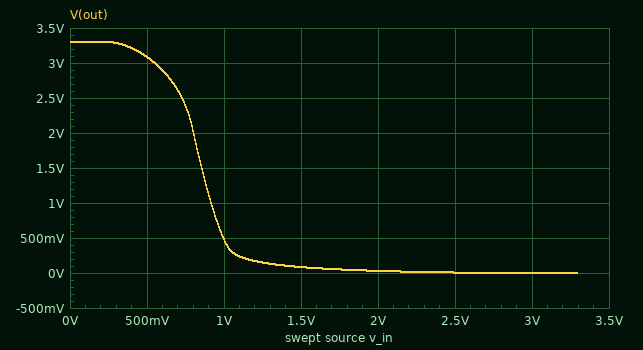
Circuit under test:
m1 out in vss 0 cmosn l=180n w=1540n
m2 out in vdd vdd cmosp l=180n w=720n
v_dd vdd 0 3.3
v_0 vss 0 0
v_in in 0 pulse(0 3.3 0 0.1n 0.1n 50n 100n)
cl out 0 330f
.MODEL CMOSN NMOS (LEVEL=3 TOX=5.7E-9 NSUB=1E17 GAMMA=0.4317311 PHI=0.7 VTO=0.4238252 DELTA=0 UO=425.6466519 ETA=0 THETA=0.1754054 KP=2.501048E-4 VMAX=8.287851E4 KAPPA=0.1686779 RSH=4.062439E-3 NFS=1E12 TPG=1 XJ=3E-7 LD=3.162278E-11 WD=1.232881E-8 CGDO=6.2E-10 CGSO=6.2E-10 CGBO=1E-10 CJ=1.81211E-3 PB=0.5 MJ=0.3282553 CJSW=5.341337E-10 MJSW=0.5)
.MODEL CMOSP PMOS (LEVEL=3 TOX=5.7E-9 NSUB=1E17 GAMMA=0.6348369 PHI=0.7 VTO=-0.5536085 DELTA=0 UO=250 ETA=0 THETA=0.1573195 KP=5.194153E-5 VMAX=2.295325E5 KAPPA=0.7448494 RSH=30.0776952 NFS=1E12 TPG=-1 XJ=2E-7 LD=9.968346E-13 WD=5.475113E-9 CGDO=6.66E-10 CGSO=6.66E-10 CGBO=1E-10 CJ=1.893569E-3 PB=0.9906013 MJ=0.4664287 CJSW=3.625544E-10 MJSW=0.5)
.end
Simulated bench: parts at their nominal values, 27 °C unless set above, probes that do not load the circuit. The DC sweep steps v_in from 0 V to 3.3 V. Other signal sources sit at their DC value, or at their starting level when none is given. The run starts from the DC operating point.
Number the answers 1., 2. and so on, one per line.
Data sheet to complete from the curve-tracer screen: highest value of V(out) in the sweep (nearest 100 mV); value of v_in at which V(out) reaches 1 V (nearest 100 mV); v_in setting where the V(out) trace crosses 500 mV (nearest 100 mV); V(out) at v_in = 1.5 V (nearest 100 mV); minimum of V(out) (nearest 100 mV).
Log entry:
1. 3.3 V
2. 900 mV
3. 1.0 V
4. 100 mV
5. 0 V
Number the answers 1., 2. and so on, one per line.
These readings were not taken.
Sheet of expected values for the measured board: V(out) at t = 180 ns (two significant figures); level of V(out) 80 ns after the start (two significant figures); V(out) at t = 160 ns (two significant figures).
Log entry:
1. 3.3 V
2. 3.3 V
3. 3.3 V
